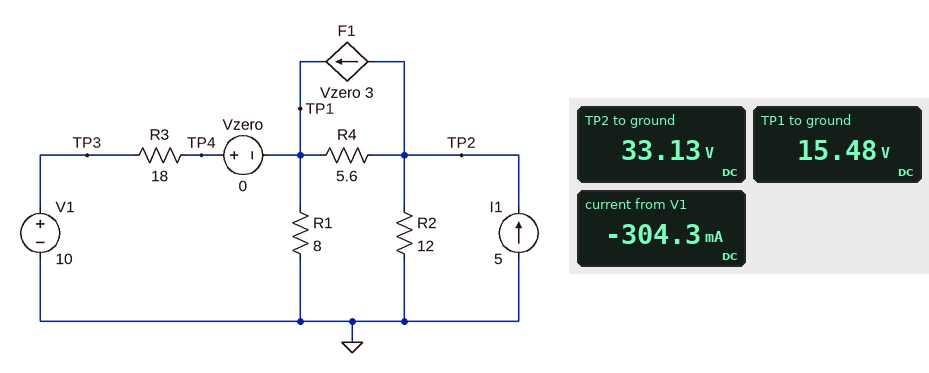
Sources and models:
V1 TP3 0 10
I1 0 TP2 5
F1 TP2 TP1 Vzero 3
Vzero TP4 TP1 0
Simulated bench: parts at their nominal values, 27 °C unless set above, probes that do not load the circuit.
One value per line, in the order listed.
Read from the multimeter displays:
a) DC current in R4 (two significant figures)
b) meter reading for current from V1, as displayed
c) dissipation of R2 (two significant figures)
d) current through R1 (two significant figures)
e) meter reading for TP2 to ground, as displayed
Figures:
3.2 A
-304.3 mA
91 W
1.9 A
33.13 V
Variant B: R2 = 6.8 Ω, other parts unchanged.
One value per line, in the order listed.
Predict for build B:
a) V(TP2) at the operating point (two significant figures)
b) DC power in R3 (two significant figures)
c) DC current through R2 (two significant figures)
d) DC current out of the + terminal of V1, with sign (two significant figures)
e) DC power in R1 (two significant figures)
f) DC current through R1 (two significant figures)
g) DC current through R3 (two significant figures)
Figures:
23 V
230 mW
3.4 A
-110 mA
18 W
1.5 A
110 mA
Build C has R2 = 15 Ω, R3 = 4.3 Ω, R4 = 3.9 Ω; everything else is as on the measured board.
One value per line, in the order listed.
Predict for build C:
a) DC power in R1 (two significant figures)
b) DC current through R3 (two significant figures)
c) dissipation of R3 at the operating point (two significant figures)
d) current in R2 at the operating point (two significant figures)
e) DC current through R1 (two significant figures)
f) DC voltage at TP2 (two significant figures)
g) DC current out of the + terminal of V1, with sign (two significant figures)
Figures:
24 W
920 mA
3.6 W
2.3 A
1.7 A
35 V
-920 mA
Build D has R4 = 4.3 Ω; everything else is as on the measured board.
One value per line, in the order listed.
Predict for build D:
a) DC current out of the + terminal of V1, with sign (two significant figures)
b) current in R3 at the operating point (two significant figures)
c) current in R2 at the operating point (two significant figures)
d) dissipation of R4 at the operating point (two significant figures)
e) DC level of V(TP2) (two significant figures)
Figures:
-350 mA
350 mA
2.6 A
51 W
31 V
